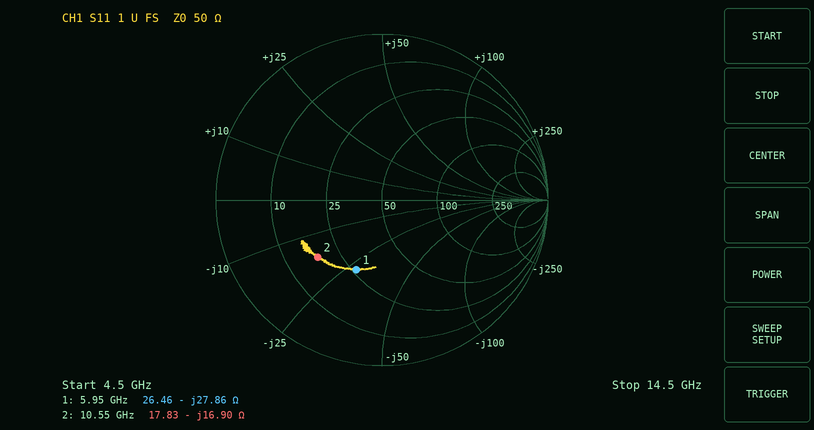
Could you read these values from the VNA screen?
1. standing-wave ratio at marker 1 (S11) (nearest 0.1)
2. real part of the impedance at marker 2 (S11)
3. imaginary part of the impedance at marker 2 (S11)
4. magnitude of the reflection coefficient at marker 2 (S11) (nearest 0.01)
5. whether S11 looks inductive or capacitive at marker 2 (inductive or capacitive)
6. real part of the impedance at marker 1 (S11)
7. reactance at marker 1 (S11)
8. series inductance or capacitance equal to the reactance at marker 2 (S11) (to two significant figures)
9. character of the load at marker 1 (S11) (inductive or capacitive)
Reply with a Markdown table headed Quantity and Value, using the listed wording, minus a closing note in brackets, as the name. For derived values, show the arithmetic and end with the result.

| Quantity | Value |
|---|---|
| standing-wave ratio at marker 1 (S11) | 2.6 |
| real part of the impedance at marker 2 | 17.83 Ω |
| imaginary part of the impedance at marker 2 | -16.90 Ω |
| magnitude of the reflection coefficient at marker 2 (S11) | 0.52 |
| whether S11 looks inductive or capacitive at marker 2 | capacitive |
| real part of the impedance at marker 1 | 26.46 Ω |
| reactance at marker 1 | -27.86 Ω |
| series inductance or capacitance equal to the reactance at marker 2 (S11) | C = 1/(2π × 10.55 GHz × 16.9 Ω) ≈ 893 fF, so 890 fF to two significant figures |
| character of the load at marker 1 (S11) | capacitive |
